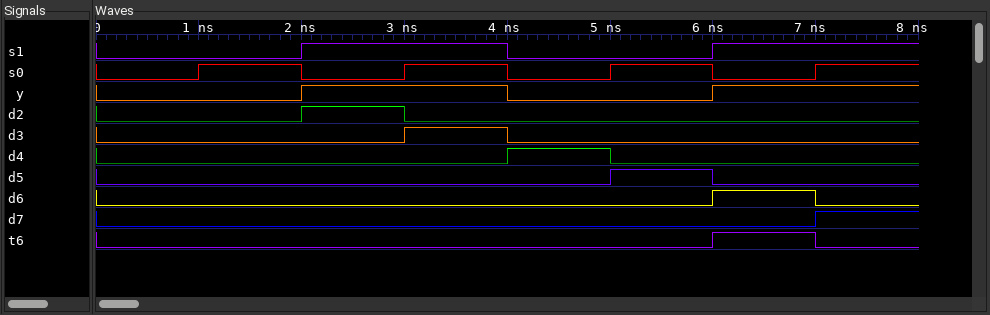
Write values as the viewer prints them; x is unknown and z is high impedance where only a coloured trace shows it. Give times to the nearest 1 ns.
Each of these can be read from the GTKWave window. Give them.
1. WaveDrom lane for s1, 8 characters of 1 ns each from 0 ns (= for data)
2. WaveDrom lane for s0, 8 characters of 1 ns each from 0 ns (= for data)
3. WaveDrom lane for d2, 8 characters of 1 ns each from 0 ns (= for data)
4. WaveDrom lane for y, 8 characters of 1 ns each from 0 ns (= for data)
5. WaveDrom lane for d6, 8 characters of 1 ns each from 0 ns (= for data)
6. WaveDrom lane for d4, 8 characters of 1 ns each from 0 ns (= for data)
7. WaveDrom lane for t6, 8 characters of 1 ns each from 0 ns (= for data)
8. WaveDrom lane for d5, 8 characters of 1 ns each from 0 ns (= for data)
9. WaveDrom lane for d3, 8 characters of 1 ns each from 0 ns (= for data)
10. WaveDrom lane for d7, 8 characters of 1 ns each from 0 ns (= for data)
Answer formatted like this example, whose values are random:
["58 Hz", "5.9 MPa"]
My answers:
["{name: 's1', wave: '0.1.0.1.'}", "{name: 's0', wave: '01010101'}", "{name: 'd2', wave: '0.10....'}", "{name: 'y', wave: '0.1.0.1.'}", "{name: 'd6', wave: '0.....10'}", "{name: 'd4', wave: '0...10..'}", "{name: 't6', wave: '0.....10'}", "{name: 'd5', wave: '0....10.'}", "{name: 'd3', wave: '0..10...'}", "{name: 'd7', wave: '0......1'}"]
